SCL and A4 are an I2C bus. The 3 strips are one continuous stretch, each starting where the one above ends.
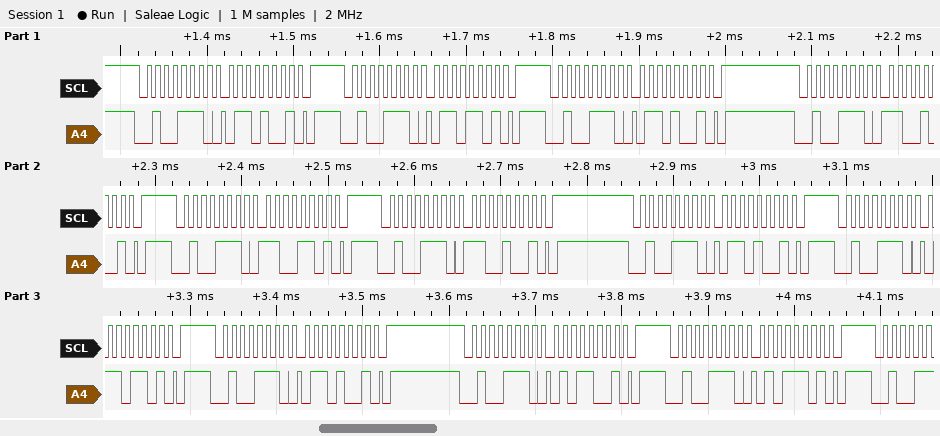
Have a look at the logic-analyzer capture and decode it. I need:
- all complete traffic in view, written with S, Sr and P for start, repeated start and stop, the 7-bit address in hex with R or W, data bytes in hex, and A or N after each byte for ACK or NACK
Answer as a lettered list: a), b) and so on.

a) S 27W A 69 A P S 27W A 6D A P S 27W A 69 A P S 27W A C9 A P S 27W A CD A P S 27W A C9 A P S 27W A 69 A P S 27W A 6D A P S 27W A 69 A P S 27W A 59 A P S 27W A 5D A P
